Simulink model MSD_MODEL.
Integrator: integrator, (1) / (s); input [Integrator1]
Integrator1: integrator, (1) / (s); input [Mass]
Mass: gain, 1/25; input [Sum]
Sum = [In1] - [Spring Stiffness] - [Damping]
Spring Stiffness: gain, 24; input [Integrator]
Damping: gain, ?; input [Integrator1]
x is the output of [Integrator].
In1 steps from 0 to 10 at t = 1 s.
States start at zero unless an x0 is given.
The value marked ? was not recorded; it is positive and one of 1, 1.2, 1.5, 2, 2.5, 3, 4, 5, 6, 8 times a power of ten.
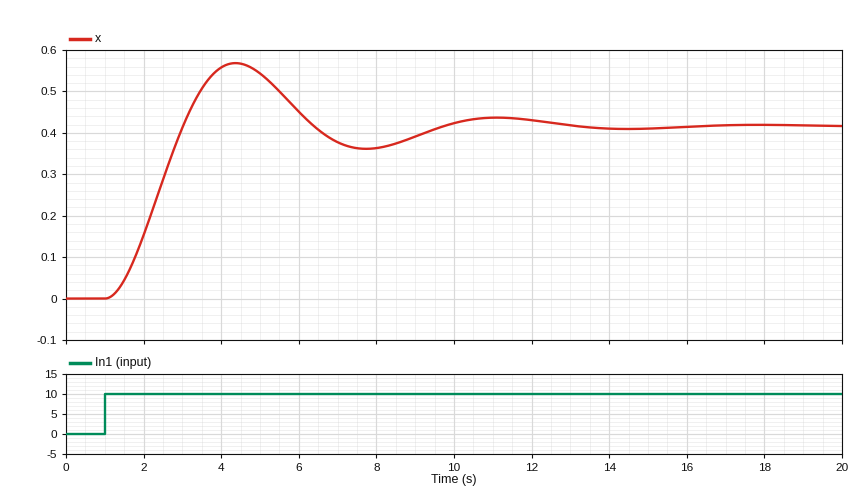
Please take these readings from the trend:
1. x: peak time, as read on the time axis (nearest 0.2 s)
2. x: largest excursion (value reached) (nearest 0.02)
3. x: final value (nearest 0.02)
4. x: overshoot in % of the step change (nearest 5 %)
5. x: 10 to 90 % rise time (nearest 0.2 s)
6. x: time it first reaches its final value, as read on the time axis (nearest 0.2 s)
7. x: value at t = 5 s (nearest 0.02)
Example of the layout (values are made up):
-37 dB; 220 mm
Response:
4.4 s; 0.56; 0.42; 35 %; 1.4 s; 3.0 s; 0.54
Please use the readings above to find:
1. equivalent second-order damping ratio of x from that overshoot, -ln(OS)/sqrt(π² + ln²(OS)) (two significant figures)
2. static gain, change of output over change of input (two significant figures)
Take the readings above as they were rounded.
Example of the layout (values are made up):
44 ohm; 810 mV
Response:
0.32; 0.042
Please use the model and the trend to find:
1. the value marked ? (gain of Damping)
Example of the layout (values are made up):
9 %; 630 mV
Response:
15
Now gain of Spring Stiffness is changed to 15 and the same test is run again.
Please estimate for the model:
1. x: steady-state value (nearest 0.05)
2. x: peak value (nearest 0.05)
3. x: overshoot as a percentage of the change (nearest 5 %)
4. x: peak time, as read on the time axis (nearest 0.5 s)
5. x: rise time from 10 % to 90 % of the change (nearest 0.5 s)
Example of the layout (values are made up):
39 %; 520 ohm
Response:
0.65; 0.85; 25 %; 5.5 s; 2.0 s
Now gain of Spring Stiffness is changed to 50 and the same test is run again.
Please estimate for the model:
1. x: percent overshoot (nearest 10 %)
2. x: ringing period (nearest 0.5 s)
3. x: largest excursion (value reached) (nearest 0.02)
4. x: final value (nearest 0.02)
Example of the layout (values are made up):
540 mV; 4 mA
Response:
50 %; 4.5 s; 0.30; 0.20
